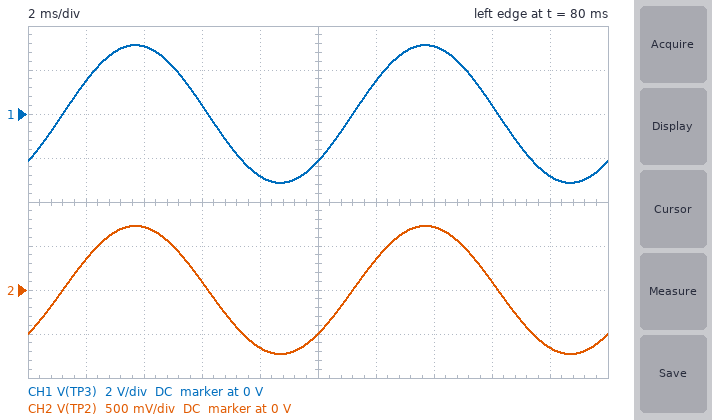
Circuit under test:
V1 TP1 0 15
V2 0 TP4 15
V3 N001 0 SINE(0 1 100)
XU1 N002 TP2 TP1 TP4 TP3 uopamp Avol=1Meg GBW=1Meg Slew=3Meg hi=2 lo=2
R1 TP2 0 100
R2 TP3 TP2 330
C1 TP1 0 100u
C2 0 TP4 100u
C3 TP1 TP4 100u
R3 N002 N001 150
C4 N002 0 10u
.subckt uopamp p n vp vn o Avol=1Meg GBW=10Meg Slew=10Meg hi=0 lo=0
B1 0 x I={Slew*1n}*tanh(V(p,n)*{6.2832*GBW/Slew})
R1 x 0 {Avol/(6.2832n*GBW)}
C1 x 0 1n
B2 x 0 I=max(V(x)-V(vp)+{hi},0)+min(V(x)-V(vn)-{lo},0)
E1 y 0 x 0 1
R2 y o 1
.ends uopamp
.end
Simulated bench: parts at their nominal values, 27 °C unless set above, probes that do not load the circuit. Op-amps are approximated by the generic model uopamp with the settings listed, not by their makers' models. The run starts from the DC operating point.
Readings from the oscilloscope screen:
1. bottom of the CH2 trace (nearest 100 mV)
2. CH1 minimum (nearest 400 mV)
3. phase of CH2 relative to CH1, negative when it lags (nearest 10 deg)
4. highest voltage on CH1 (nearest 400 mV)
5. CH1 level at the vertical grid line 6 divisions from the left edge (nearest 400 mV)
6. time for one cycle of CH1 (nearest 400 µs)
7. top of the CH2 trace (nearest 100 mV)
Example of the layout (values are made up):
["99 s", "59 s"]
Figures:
["-700 mV", "-3.2 V", "0 deg", "3.2 V", "1.6 V", "10.0 ms", "700 mV"]
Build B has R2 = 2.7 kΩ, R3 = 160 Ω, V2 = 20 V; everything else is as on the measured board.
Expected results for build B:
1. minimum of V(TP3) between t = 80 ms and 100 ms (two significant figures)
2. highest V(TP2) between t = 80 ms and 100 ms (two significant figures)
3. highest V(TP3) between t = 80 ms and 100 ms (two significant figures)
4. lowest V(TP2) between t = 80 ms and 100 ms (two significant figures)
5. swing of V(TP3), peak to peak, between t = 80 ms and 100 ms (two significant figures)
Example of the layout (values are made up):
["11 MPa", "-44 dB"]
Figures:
["-18 V", "460 mV", "13 V", "-640 mV", "31 V"]
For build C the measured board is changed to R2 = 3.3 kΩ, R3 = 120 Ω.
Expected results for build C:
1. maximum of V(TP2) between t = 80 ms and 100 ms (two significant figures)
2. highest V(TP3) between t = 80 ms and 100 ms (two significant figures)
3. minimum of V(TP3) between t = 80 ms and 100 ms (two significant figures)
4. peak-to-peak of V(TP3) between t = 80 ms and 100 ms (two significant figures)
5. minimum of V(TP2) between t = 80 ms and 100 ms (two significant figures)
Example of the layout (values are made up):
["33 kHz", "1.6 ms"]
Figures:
["380 mV", "13 V", "-13 V", "26 V", "-380 mV"]
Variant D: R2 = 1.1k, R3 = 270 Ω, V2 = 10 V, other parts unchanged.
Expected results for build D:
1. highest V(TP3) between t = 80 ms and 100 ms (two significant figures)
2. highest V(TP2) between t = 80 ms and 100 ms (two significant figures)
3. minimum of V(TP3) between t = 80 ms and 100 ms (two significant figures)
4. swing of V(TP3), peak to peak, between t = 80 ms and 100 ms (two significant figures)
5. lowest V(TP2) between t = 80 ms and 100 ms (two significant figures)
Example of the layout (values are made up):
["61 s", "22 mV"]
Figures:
["6.1 V", "510 mV", "-6.1 V", "12 V", "-510 mV"]
